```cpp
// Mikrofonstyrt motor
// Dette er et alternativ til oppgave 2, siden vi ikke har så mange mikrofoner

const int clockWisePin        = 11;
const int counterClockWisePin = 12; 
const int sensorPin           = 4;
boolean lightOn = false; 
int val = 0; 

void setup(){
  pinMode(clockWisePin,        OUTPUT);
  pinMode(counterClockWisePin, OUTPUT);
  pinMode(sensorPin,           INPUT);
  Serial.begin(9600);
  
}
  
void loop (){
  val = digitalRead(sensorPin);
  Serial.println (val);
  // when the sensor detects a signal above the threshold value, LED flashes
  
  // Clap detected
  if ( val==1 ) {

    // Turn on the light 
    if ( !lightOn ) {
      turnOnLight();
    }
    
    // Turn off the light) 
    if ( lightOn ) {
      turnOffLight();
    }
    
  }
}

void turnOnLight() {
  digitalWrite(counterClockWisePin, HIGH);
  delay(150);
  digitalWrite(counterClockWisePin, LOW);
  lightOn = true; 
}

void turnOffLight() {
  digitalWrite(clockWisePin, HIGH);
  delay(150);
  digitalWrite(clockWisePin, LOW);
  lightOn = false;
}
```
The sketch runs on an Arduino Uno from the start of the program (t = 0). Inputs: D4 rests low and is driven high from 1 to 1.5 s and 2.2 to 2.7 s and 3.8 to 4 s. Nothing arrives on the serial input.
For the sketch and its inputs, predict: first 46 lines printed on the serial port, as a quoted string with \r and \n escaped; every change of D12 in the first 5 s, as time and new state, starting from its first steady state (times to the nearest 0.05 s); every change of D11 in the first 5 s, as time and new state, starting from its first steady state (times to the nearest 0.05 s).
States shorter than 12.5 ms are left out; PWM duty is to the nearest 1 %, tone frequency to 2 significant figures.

"0\r\n0\r\n0\r\n0\r\n0\r\n0\r\n0\r\n0\r\n0\r\n0\r\n0\r\n0\r\n0\r\n0\r\n0\r\n0\r\n0\r\n0\r\n0\r\n0\r\n0\r\n0\r\n0\r\n0\r\n0\r\n0\r\n0\r\n0\r\n0\r\n0\r\n0\r\n0\r\n0\r\n0\r\n0\r\n0\r\n0\r\n0\r\n0\r\n0\r\n0\r\n0\r\n0\r\n0\r\n0\r\n0\r\n"
0 s low; 1 s high; 1.15 s low; 1.3 s high; 1.45 s low; 2.2 s high; 2.35 s low; 2.5 s high; 2.65 s low; 3.8 s high; 3.95 s low
0 s low; 1.15 s high; 1.3 s low; 1.45 s high; 1.6 s low; 2.35 s high; 2.5 s low; 2.65 s high; 2.8 s low; 3.95 s high; 4.1 s low
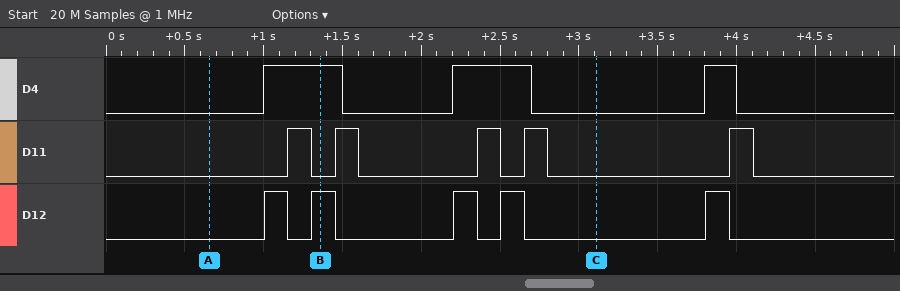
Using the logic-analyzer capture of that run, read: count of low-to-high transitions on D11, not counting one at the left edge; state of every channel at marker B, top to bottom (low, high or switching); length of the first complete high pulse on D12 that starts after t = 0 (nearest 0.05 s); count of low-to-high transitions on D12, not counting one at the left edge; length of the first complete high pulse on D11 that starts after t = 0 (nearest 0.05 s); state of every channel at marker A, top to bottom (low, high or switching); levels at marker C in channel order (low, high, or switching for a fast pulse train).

5
D4 high, D11 low, D12 high
0.15 s
5
0.15 s
D4 low, D11 low, D12 low
D4 low, D11 low, D12 low
